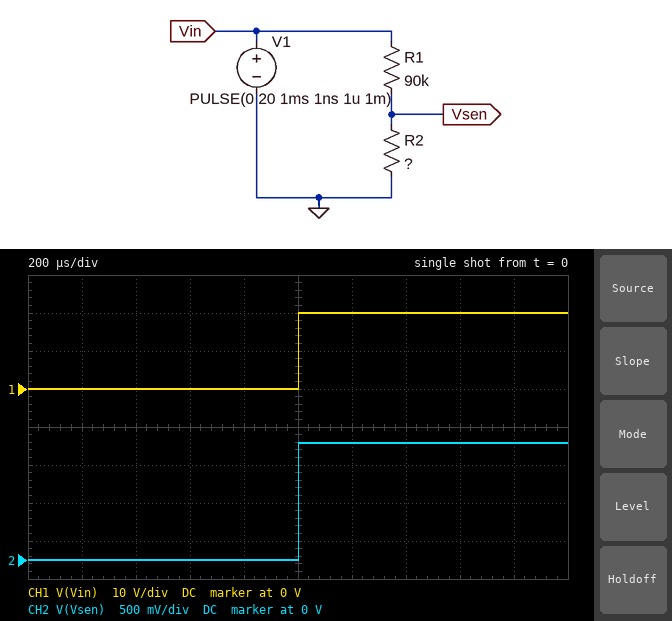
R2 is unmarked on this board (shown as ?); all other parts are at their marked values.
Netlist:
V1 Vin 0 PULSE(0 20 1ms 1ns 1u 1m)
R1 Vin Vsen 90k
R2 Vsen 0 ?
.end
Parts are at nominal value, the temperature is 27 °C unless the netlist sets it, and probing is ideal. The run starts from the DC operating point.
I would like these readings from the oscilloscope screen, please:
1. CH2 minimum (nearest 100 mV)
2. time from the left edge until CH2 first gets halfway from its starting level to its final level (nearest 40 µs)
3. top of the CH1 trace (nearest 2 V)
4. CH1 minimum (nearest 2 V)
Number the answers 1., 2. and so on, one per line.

1. 0 V
2. 1.00 ms
3. 20 V
4. 0 V
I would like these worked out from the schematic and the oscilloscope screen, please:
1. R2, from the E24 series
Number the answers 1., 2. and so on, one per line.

1. 7.5 kΩ
